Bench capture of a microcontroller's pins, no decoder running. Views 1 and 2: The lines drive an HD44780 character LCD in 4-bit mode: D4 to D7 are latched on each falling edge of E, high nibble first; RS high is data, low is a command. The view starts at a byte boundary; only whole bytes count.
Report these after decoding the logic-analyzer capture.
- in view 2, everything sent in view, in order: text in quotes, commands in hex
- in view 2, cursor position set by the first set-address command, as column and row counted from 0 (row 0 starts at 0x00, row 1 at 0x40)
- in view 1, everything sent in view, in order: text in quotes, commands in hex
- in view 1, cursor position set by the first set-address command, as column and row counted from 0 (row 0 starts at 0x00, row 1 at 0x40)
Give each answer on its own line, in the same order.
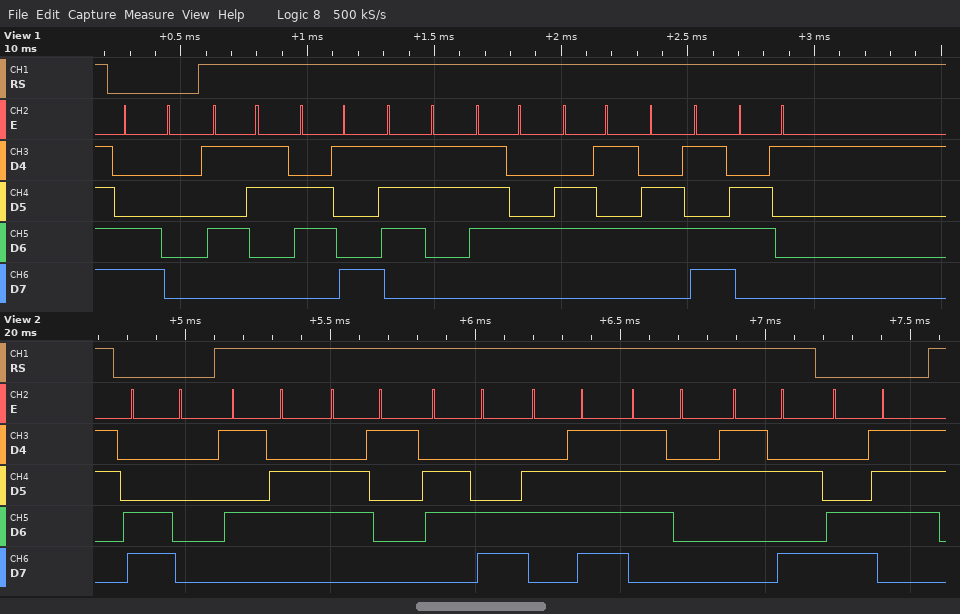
0xC0 "Valor:" 0xC7
column 0, row 1
0xC0 "Sistema"
column 0, row 1
